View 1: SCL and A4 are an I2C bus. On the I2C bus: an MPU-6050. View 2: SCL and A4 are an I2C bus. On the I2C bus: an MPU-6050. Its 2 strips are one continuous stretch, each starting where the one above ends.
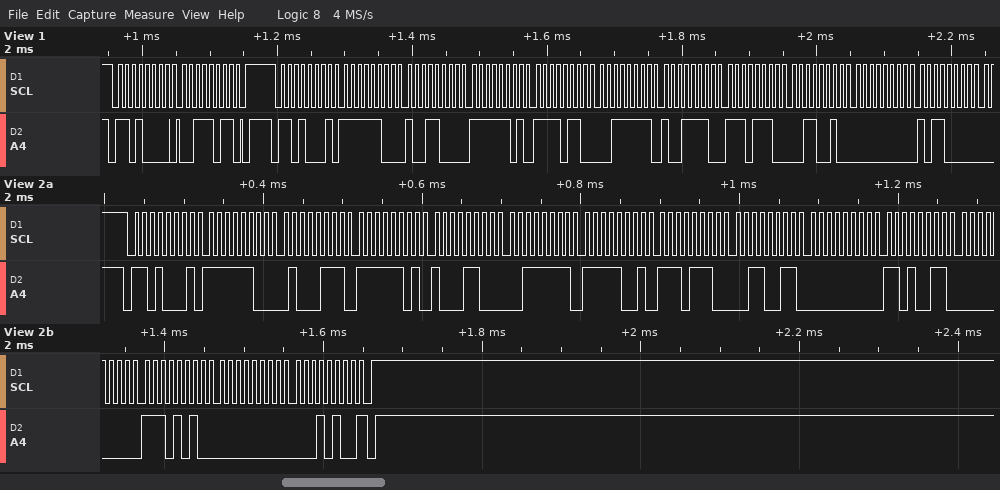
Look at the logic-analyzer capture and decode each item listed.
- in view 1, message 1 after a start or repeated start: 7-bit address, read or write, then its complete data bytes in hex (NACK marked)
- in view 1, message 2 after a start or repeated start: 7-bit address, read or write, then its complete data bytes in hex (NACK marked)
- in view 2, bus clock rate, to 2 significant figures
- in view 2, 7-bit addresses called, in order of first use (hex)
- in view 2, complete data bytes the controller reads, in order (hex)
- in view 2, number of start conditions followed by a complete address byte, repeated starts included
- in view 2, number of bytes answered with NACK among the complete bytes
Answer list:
0x68 write: 3B
0x68 read: FC 98 FD F6 3F 9E EE 32 00 B0
100 kHz
0x68
FC 47 FD 8C 3F F9 EE 33 00 D3 00 EA 00 14
1
1
